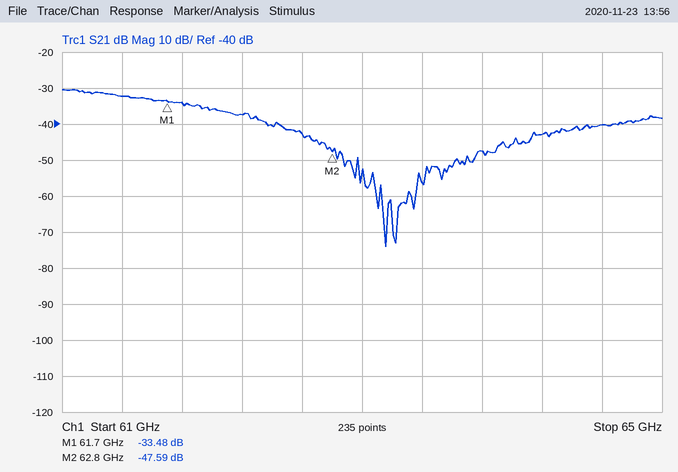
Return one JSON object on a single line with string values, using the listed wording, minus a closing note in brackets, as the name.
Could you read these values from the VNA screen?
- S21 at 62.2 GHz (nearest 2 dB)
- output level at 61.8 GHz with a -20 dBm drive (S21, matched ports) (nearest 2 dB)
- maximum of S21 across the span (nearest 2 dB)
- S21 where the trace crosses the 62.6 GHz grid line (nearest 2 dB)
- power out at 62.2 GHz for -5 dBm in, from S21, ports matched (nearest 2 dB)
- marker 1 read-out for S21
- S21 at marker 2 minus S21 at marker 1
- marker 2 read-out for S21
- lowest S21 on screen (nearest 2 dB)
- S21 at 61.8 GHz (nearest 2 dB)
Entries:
{"S21 at 62.2 GHz": "-38 dB", "output level at 61.8 GHz with a -20 dBm drive (S21, matched ports)": "-54 dBm", "maximum of S21 across the span": "-30 dB", "S21 where the trace crosses the 62.6 GHz grid line": "-42 dB", "power out at 62.2 GHz for -5 dBm in, from S21, ports matched": "-42 dBm", "marker 1 read-out for S21": "-33.48 dB", "S21 at marker 2 minus S21 at marker 1": "-14.11 dB", "marker 2 read-out for S21": "-47.59 dB", "lowest S21 on screen": "-74 dB", "S21 at 61.8 GHz": "-34 dB"}
